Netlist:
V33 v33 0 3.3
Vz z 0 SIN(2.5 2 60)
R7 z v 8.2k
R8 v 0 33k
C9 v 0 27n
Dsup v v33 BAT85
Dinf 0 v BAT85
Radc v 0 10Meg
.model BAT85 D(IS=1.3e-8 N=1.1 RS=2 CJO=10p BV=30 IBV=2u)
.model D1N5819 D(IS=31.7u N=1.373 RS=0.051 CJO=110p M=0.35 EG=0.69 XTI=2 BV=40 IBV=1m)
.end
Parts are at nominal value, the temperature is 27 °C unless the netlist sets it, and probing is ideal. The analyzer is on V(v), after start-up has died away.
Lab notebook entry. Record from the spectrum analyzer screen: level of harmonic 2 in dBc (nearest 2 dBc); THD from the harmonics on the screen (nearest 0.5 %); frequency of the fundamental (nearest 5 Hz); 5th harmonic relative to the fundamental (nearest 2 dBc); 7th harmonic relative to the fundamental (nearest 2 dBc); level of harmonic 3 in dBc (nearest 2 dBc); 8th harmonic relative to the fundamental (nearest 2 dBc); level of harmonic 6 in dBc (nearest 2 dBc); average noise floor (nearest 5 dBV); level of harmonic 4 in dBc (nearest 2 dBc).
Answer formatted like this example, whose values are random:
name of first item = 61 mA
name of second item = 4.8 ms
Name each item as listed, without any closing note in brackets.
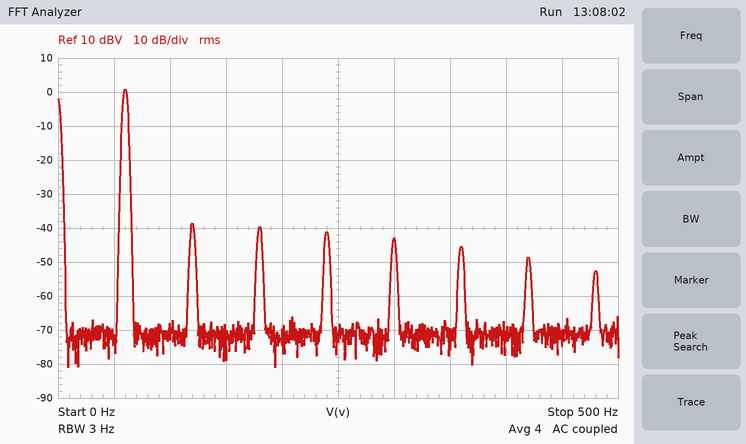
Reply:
level of harmonic 2 in dBc = -40 dBc
THD from the harmonics on the screen = 2.0 %
frequency of the fundamental = 60 Hz
5th harmonic relative to the fundamental = -44 dBc
7th harmonic relative to the fundamental = -50 dBc
level of harmonic 3 in dBc = -40 dBc
8th harmonic relative to the fundamental = -54 dBc
level of harmonic 6 in dBc = -46 dBc
average noise floor = -70 dBV
level of harmonic 4 in dBc = -42 dBc
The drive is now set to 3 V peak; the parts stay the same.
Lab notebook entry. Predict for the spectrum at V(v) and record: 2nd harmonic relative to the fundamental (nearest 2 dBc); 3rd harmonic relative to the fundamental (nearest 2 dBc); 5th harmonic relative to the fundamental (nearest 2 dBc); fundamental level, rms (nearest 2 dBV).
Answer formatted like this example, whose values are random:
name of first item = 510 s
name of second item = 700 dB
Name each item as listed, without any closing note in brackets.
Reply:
2nd harmonic relative to the fundamental = -20 dBc
3rd harmonic relative to the fundamental = -22 dBc
5th harmonic relative to the fundamental = -38 dBc
fundamental level, rms = 4 dBV
